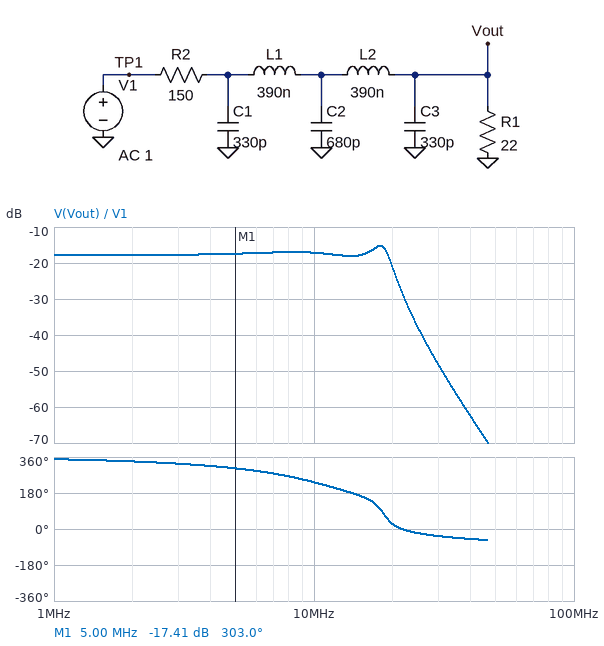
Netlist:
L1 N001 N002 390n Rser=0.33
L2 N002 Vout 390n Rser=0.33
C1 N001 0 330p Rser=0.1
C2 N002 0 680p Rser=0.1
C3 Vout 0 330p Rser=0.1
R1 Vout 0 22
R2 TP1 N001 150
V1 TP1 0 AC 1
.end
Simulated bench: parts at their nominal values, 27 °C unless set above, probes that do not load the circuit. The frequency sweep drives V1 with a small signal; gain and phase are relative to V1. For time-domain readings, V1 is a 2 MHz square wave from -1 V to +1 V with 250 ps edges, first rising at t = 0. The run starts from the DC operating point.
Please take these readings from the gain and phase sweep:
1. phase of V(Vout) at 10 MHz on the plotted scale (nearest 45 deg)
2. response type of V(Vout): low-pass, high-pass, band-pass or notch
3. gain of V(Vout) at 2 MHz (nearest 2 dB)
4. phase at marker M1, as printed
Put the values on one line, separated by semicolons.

225 deg; low-pass; -18 dB; 303.0 deg
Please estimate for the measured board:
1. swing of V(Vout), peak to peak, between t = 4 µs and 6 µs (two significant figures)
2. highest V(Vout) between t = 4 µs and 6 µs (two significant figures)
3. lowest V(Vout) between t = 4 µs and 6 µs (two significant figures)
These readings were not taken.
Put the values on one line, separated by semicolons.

380 mV; 190 mV; -190 mV
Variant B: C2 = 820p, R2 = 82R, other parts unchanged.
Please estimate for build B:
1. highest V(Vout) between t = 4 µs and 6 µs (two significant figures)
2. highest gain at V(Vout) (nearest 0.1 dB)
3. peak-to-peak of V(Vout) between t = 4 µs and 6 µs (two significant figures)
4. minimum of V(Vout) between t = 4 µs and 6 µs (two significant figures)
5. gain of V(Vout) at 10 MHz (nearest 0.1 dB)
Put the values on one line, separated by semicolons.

280 mV; -13.2 dB; 570 mV; -280 mV; -13.5 dB
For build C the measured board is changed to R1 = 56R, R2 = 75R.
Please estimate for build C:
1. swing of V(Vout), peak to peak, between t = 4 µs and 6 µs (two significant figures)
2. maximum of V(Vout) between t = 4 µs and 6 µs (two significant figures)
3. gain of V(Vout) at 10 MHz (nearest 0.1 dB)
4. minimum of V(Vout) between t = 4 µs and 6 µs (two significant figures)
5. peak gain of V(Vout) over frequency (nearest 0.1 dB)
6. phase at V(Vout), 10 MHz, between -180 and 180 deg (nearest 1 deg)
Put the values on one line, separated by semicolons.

870 mV; 430 mV; -9.7 dB; -430 mV; -7.4 dB; -115 deg
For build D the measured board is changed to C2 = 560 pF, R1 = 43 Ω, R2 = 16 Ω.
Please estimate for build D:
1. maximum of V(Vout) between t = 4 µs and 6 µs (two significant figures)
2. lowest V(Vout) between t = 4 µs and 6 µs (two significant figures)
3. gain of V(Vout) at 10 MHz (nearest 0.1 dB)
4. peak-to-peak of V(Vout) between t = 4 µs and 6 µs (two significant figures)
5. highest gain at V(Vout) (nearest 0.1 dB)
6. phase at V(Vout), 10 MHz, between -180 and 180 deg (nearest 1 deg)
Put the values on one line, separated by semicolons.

1.0 V; -1.0 V; -2.2 dB; 2.1 V; -1.9 dB; -118 deg
